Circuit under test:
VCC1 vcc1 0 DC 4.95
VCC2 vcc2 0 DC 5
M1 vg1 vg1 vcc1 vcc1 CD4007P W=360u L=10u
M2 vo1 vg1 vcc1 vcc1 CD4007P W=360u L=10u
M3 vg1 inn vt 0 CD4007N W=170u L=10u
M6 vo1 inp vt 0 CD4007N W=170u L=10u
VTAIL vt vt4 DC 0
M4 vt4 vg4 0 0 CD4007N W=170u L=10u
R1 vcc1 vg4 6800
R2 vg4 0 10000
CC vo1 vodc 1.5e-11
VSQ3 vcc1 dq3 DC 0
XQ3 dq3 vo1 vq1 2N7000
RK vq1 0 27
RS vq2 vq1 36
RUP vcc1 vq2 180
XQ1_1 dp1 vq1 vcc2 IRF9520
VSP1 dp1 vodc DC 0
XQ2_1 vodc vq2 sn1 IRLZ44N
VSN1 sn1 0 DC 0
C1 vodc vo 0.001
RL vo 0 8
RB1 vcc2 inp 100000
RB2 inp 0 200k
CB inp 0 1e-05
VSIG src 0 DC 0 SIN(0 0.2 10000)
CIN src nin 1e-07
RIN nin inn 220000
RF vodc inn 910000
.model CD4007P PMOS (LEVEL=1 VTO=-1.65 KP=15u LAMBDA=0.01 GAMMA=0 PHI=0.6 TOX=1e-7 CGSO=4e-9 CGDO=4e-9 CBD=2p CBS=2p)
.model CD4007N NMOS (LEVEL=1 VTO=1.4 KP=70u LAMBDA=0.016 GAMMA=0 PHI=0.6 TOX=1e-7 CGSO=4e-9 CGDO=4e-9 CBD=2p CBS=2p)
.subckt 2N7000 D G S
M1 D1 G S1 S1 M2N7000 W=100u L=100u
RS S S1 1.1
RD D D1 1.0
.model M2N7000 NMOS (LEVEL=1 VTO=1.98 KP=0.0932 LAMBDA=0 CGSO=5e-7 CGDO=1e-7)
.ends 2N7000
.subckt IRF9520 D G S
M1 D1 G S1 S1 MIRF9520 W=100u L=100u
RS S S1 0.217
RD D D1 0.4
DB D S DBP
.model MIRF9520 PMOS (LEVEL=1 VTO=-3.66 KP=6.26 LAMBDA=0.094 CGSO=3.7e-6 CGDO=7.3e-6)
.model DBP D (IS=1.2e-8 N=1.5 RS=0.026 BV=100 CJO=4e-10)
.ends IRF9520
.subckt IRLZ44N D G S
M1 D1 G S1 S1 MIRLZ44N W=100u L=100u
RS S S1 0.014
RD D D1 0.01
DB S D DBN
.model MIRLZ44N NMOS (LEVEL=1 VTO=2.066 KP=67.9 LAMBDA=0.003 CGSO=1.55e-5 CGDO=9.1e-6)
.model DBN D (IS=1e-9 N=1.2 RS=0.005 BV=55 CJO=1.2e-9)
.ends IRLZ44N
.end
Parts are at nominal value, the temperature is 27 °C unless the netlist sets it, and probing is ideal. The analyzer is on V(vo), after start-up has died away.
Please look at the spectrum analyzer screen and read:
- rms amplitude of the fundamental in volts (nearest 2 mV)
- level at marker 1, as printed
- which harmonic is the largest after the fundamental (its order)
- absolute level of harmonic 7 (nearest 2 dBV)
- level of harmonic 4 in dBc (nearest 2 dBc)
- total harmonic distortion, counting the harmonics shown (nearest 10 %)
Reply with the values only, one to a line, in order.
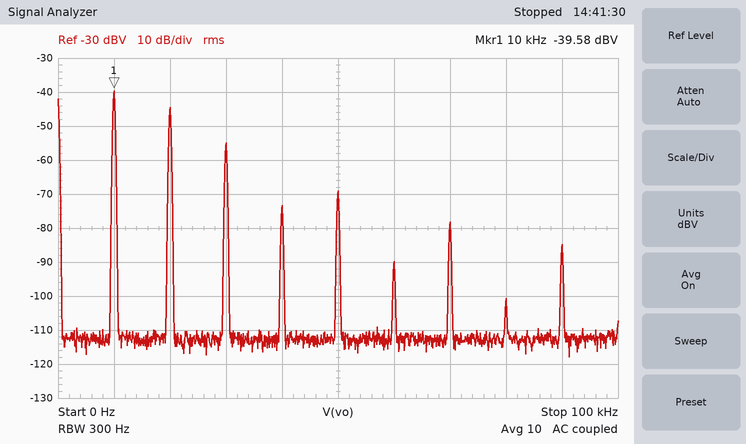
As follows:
10 mV
-39.58 dBV
2
-78 dBV
-34 dBc
60 %
